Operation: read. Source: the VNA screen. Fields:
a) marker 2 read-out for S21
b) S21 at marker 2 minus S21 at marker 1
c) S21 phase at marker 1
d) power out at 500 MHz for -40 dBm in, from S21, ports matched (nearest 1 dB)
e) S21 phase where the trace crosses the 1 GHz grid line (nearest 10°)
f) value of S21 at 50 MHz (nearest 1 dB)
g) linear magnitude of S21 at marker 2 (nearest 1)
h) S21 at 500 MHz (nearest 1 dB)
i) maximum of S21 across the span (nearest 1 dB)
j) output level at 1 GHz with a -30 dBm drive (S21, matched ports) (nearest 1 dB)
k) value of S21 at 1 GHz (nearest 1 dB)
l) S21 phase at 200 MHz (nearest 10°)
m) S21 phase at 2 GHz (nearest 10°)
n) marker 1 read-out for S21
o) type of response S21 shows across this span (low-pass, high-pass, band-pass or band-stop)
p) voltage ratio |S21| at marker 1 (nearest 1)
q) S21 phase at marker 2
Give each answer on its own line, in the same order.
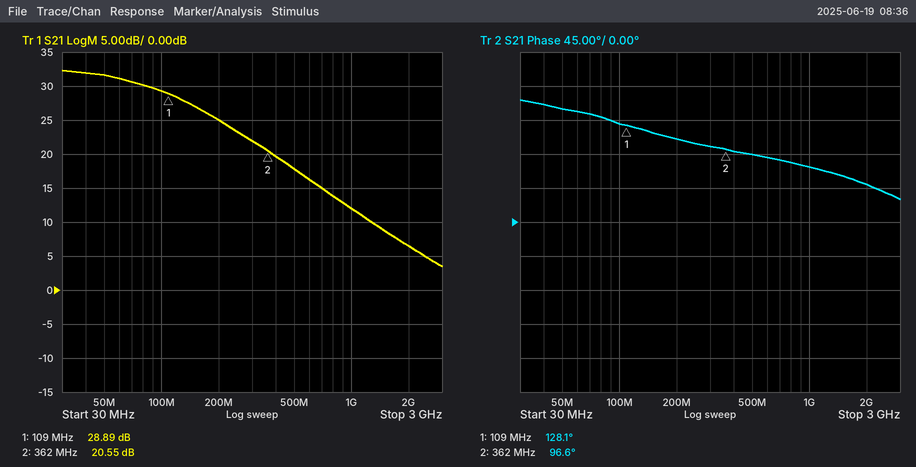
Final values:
20.55 dB
-8.34 dB
128.1°
-22 dBm
70°
32 dB
11
18 dB
32 dB
-18 dBm
12 dB
110°
50°
28.89 dB
low-pass
28
96.6°
